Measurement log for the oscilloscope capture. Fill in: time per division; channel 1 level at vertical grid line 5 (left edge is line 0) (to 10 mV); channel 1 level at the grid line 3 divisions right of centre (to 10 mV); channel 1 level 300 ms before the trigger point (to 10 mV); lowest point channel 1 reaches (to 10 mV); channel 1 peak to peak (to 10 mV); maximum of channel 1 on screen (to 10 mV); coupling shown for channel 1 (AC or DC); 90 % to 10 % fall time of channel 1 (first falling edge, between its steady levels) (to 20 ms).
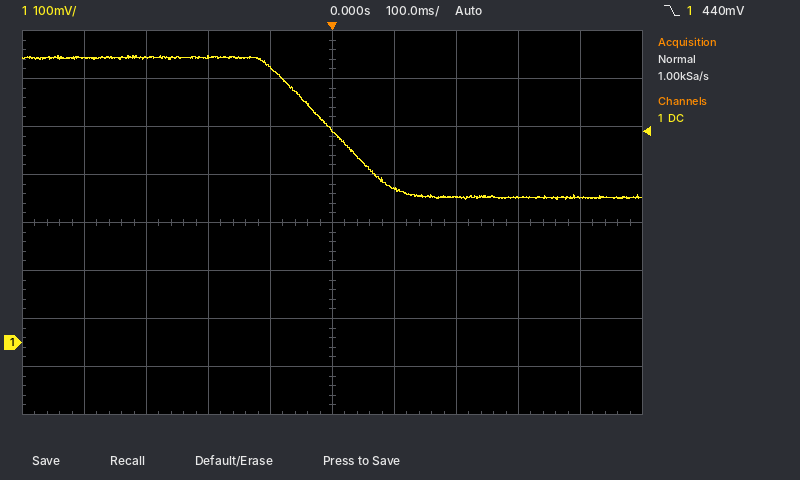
100 ms
440 mV
300 mV
590 mV
300 mV
300 mV
600 mV
DC
180 ms
